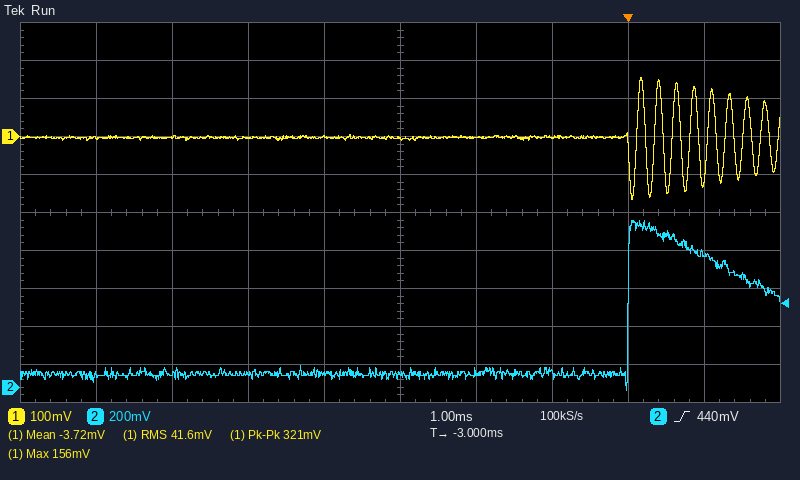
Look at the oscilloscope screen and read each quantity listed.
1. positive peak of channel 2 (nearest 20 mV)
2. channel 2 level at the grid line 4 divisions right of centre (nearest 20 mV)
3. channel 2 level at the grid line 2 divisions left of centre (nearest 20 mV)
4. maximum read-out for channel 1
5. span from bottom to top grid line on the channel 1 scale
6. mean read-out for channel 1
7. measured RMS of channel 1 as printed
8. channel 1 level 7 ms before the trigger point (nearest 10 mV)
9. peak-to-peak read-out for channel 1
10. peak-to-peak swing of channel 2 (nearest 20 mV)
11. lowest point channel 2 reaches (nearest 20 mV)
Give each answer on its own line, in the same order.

880 mV
700 mV
60 mV
156 mV
1 V
-3.72 mV
41.6 mV
0 mV
321 mV
900 mV
-20 mV
